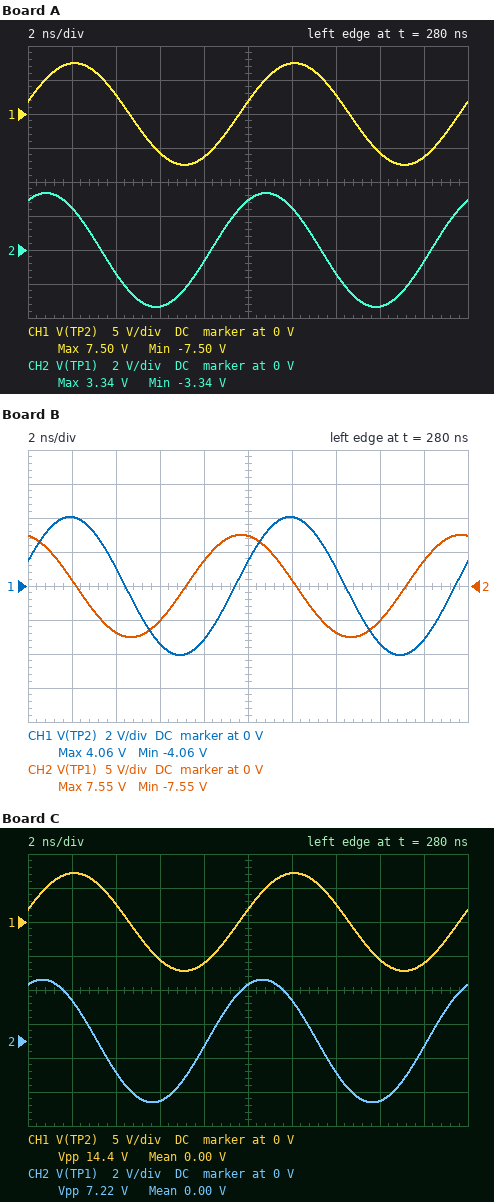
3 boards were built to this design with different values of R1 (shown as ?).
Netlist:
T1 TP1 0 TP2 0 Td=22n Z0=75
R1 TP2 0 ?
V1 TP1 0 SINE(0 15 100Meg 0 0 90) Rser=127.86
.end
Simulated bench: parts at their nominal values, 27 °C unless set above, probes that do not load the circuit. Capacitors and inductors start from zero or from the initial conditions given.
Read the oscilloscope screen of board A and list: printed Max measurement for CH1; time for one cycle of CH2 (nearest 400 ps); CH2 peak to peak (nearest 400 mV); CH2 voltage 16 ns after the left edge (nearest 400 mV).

7.50 V
10.0 ns
6.8 V
-3.2 V
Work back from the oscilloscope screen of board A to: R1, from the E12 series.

220 Ω
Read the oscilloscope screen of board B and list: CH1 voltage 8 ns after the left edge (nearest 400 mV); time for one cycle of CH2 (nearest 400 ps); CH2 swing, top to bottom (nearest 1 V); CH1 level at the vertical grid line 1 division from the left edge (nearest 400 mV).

-3.2 V
10.0 ns
15 V
4.0 V
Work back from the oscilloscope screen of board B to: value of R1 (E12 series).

39 Ω
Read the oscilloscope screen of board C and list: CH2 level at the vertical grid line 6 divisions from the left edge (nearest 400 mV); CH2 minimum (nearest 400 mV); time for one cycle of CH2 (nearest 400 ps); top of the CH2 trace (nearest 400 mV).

2.4 V
-3.6 V
10.0 ns
3.6 V
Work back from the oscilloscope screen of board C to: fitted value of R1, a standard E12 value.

180 Ω
